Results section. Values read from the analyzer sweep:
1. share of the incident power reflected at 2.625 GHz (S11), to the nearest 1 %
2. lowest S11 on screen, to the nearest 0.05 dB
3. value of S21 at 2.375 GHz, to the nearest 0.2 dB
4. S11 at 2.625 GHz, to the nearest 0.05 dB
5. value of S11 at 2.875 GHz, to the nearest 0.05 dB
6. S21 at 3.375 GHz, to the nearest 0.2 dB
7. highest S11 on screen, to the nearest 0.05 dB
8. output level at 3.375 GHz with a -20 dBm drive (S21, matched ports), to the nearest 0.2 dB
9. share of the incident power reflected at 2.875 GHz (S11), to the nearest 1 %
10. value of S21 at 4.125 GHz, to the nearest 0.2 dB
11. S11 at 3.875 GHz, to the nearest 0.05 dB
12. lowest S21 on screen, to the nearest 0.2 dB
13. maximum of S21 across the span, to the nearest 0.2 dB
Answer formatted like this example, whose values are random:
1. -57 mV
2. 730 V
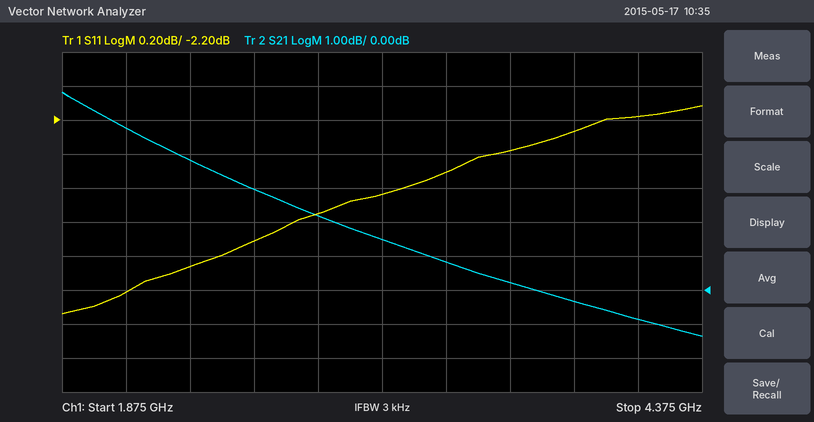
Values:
1. 51 %
2. -3.35 dB
3. 3.8 dB
4. -2.90 dB
5. -2.75 dB
6. 0.8 dB
7. -2.10 dB
8. -19.2 dBm
9. 53 %
10. -0.8 dB
11. -2.25 dB
12. -1.4 dB
13. 5.8 dB
